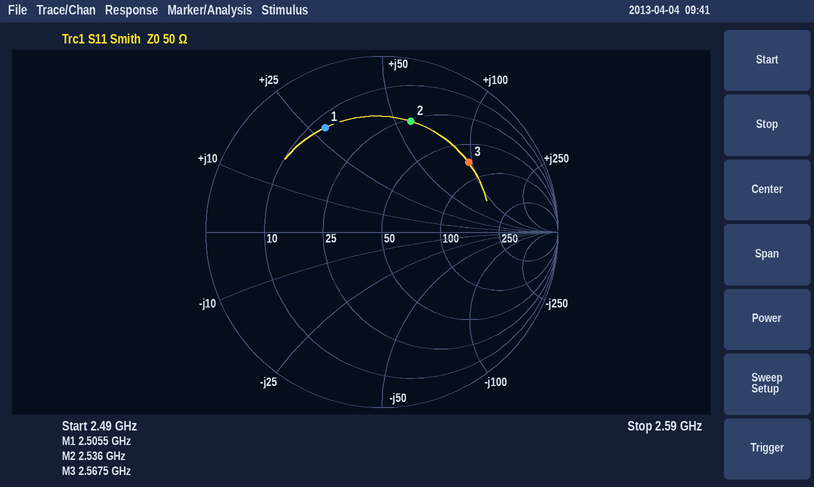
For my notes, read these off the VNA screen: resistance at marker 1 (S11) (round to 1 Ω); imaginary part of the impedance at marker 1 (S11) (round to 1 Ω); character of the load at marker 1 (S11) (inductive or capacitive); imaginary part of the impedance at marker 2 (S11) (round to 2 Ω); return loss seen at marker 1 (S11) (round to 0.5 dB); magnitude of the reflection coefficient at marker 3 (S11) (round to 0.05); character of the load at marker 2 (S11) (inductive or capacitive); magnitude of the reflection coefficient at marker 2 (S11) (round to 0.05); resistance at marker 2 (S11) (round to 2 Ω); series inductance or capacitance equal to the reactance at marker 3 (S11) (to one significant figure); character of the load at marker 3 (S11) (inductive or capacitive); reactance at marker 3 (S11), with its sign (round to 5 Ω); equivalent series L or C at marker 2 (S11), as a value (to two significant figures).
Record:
13 Ω
+28 Ω
inductive
+58 Ω
3.5 dB
0.65
inductive
0.65
26 Ω
6 nH
inductive
+95 Ω
3.6 nH
